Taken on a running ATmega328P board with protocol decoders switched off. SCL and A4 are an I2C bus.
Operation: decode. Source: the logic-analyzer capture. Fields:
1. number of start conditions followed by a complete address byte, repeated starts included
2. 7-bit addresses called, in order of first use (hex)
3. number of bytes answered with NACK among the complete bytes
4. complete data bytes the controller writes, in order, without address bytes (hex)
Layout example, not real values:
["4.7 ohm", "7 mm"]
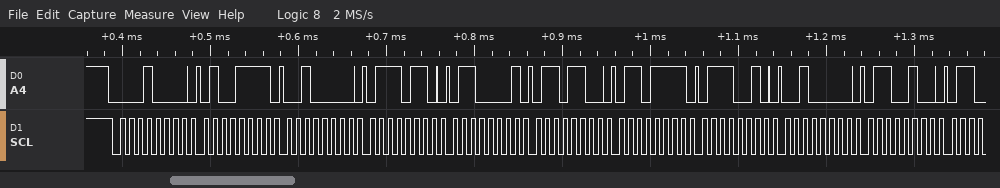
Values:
["1", "0x08", "0", "4F 20 76 61 6C 6F 72 20 64"]
